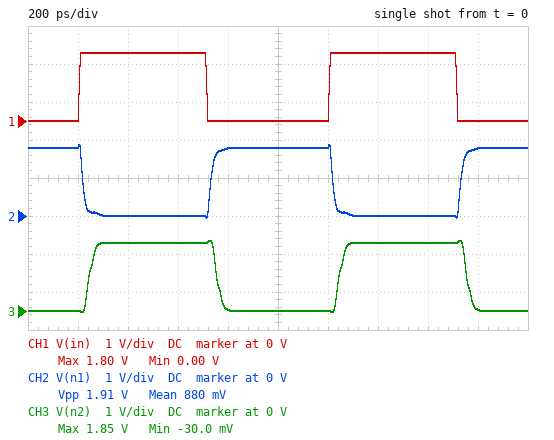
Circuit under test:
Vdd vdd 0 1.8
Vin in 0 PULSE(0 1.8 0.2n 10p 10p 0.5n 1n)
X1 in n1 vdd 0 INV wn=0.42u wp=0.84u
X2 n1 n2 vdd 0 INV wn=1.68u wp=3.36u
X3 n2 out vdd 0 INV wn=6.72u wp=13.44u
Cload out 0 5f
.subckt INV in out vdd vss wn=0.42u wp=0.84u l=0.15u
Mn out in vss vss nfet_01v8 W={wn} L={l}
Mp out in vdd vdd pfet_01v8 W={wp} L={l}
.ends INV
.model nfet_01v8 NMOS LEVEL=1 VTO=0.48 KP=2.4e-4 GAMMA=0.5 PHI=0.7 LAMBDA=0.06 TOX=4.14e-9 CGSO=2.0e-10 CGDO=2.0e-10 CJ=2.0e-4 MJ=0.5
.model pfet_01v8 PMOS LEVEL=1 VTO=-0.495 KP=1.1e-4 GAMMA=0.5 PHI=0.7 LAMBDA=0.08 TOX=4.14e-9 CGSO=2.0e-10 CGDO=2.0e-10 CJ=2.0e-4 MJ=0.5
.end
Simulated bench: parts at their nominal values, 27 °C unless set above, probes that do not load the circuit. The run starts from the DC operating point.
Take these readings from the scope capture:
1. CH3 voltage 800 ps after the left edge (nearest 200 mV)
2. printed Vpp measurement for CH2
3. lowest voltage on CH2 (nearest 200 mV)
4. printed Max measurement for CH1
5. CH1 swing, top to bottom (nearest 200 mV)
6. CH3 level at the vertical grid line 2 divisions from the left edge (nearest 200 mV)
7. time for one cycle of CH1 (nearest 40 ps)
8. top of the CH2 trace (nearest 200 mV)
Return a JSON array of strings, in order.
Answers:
["0 V", "1.91 V", "0 V", "1.80 V", "1.8 V", "1.8 V", "1.00 ns", "1.8 V"]
